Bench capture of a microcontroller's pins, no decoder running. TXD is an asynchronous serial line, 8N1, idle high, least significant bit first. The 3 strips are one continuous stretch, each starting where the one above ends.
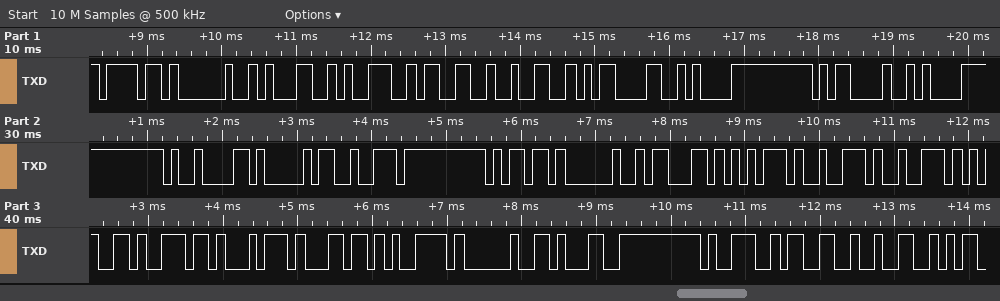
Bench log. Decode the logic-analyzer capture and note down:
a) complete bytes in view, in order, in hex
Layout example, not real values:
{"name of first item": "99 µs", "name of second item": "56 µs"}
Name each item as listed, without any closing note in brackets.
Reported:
{"complete bytes in view, in order, in hex": "6F 20 31 39 33 32 0D 0A 0D 0A 09 41 72 6D 20 63 75 72 72 65 6E 74 6C 79 20 31 39 33 32"}
